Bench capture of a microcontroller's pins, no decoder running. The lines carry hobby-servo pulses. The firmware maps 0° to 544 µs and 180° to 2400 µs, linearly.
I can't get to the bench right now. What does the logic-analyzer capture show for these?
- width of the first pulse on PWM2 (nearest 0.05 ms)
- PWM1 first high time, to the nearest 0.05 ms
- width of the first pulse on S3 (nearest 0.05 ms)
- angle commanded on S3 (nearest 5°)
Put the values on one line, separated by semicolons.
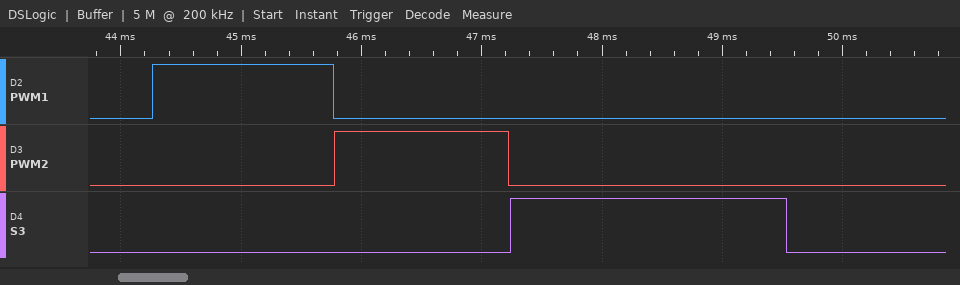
1.45 ms; 1.50 ms; 2.30 ms; 170°
